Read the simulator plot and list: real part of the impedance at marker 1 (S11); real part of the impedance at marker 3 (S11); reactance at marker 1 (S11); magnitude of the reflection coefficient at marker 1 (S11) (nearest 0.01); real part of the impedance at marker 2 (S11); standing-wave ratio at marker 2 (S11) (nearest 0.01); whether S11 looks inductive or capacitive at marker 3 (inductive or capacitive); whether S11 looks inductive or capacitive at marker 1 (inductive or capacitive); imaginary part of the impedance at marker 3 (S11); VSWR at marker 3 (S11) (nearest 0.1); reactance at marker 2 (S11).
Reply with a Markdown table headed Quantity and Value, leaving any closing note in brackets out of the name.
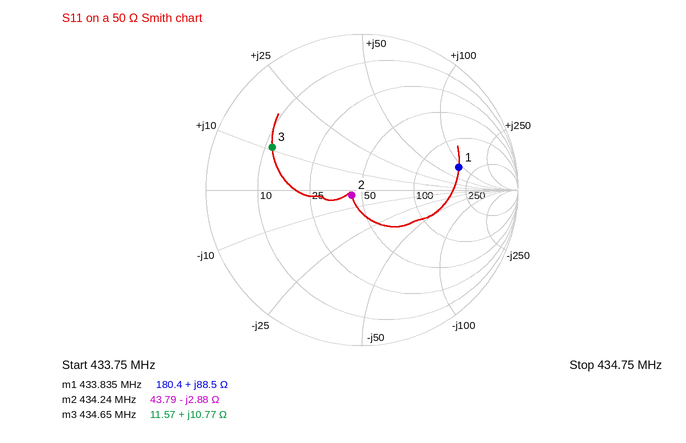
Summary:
| Quantity | Value |
|---|---|
| real part of the impedance at marker 1 | 180.4 Ω |
| real part of the impedance at marker 3 | 11.57 Ω |
| reactance at marker 1 | +88.5 Ω |
| magnitude of the reflection coefficient at marker 1 (S11) | 0.64 |
| real part of the impedance at marker 2 | 43.79 Ω |
| standing-wave ratio at marker 2 (S11) | 1.16 |
| whether S11 looks inductive or capacitive at marker 3 | inductive |
| whether S11 looks inductive or capacitive at marker 1 | inductive |
| imaginary part of the impedance at marker 3 | +10.77 Ω |
| VSWR at marker 3 (S11) | 4.5 |
| reactance at marker 2 | -2.88 Ω |
